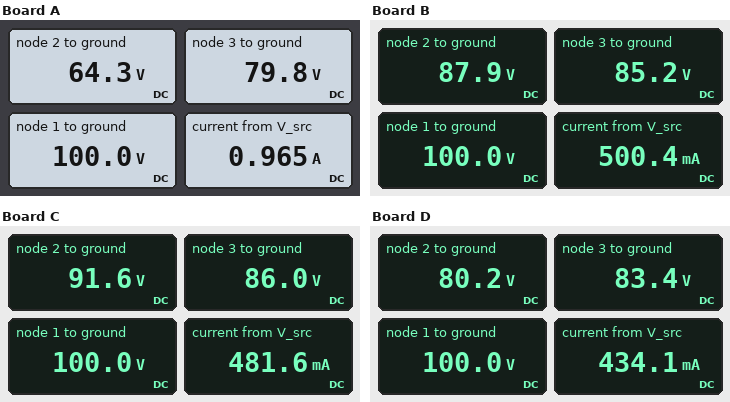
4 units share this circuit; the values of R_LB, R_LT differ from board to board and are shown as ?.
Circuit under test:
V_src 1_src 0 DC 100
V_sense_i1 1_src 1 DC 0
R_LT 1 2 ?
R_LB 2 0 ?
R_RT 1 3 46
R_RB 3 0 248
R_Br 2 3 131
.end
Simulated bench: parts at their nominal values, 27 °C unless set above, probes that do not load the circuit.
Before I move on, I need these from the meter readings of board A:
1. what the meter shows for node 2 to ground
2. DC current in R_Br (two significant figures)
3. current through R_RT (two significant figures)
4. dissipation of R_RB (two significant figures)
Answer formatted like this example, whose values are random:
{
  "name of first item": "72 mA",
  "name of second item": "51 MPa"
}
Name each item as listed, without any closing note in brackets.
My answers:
{
  "what the meter shows for node 2 to ground": "64.3 V",
  "DC current in R_Br": "120 mA",
  "current through R_RT": "440 mA",
  "dissipation of R_RB": "26 W"
}
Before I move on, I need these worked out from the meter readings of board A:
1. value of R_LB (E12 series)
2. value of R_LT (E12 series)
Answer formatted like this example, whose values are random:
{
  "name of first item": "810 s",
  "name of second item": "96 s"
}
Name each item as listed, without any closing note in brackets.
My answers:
{
  "value of R_LB": "100 Ω",
  "value of R_LT": "68 Ω"
}
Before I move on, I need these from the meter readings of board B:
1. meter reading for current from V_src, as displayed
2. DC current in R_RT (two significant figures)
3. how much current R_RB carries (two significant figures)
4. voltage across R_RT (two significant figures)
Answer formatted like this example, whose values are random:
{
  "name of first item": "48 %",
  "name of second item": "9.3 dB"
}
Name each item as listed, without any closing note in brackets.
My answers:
{
  "meter reading for current from V_src, as displayed": "500.4 mA",
  "DC current in R_RT": "320 mA",
  "how much current R_RB carries": "340 mA",
  "voltage across R_RT": "15 V"
}
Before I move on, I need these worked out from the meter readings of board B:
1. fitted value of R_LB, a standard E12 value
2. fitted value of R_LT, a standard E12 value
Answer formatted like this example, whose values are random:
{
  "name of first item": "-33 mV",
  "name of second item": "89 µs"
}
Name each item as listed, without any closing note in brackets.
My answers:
{
  "fitted value of R_LB, a standard E12 value": "560 Ω",
  "fitted value of R_LT, a standard E12 value": "68 Ω"
}
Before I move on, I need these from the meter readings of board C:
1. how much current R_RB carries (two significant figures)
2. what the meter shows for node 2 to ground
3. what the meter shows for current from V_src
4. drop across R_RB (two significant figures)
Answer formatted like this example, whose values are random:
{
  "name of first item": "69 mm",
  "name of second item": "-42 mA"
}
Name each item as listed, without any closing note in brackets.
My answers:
{
  "how much current R_RB carries": "350 mA",
  "what the meter shows for node 2 to ground": "91.6 V",
  "what the meter shows for current from V_src": "481.6 mA",
  "drop across R_RB": "86 V"
}
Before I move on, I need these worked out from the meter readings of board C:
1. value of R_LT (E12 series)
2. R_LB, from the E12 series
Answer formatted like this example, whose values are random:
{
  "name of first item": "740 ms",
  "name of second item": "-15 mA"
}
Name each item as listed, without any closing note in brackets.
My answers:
{
  "value of R_LT": "47 Ω",
  "R_LB, from the E12 series": "680 Ω"
}
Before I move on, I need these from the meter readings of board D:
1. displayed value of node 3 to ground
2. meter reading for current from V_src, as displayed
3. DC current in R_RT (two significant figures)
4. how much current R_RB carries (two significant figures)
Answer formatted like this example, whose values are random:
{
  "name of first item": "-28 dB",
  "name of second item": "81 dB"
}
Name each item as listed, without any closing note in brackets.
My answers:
{
  "displayed value of node 3 to ground": "83.4 V",
  "meter reading for current from V_src, as displayed": "434.1 mA",
  "DC current in R_RT": "360 mA",
  "how much current R_RB carries": "340 mA"
}
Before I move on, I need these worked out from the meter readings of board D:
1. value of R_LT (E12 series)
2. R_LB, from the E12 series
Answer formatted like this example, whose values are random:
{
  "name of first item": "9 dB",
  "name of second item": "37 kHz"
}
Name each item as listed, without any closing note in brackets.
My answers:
{
  "value of R_LT": "270 Ω",
  "R_LB, from the E12 series": "820 Ω"
}
